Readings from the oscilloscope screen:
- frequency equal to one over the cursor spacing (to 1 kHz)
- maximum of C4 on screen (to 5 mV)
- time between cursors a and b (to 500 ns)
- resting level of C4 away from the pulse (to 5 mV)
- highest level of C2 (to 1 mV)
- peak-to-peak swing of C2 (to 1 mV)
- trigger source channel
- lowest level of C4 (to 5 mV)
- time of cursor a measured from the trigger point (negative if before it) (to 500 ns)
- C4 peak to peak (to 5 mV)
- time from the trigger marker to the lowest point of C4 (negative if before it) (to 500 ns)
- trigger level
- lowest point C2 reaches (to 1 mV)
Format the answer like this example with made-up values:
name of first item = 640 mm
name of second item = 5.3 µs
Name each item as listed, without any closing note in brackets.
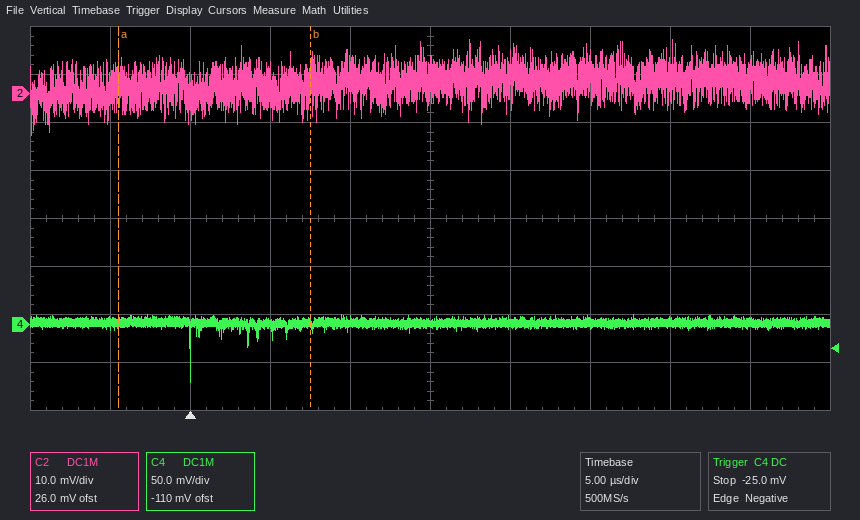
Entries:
frequency equal to one over the cursor spacing = 83 kHz
maximum of C4 on screen = 10 mV
time between cursors a and b = 12.0 µs
resting level of C4 away from the pulse = 0 mV
highest level of C2 = 11 mV
peak-to-peak swing of C2 = 20 mV
trigger source channel = C4
lowest level of C4 = -60 mV
time of cursor a measured from the trigger point (negative if before it) = -4.5 µs
C4 peak to peak = 70 mV
time from the trigger marker to the lowest point of C4 (negative if before it) = 0.0 µs
trigger level = -25.0 mV
lowest point C2 reaches = -9 mV
